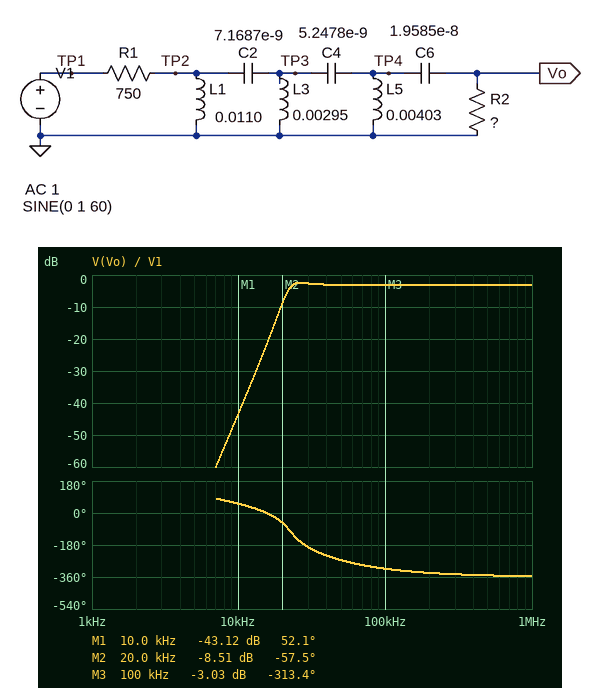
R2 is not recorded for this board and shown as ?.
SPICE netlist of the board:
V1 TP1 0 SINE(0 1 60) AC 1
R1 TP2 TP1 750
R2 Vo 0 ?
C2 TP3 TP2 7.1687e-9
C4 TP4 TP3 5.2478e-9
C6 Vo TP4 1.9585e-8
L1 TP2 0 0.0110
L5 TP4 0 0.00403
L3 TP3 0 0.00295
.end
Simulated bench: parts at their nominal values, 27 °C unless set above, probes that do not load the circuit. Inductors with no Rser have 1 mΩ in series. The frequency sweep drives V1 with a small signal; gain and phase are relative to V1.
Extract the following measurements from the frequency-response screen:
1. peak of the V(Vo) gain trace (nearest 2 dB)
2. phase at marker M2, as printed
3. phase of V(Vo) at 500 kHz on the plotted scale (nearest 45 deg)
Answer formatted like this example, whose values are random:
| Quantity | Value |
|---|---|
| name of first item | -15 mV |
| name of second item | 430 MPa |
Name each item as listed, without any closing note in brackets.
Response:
| Quantity | Value |
|---|---|
| peak of the V(Vo) gain trace | -2 dB |
| phase at marker M2, as printed | -57.5 deg |
| phase of V(Vo) at 500 kHz on the plotted scale | -360 deg |
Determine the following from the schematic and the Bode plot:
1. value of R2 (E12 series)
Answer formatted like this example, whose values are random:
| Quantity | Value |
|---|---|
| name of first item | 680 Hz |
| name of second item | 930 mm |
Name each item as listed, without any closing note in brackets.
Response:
| Quantity | Value |
|---|---|
| value of R2 | 1.8 kΩ |
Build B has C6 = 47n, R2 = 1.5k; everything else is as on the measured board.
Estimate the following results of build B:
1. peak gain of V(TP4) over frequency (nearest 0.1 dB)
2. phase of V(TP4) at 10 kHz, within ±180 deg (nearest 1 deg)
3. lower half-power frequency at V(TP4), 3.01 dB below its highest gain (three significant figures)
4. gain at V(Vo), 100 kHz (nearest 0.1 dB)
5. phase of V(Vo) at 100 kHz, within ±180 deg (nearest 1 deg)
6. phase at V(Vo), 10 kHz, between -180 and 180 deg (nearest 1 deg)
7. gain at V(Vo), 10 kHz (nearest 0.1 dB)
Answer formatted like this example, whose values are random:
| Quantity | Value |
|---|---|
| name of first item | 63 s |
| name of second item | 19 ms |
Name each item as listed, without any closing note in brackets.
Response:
| Quantity | Value |
|---|---|
| peak gain of V(TP4) over frequency | -3.1 dB |
| phase of V(TP4) at 10 kHz, within ±180 deg | 25 deg |
| lower half-power frequency at V(TP4), 3.01 dB below its highest gain | 21.5 kHz |
| gain at V(Vo), 100 kHz | -3.5 dB |
| phase of V(Vo) at 100 kHz, within ±180 deg | 45 deg |
| phase at V(Vo), 10 kHz, between -180 and 180 deg | 38 deg |
| gain at V(Vo), 10 kHz | -42.8 dB |
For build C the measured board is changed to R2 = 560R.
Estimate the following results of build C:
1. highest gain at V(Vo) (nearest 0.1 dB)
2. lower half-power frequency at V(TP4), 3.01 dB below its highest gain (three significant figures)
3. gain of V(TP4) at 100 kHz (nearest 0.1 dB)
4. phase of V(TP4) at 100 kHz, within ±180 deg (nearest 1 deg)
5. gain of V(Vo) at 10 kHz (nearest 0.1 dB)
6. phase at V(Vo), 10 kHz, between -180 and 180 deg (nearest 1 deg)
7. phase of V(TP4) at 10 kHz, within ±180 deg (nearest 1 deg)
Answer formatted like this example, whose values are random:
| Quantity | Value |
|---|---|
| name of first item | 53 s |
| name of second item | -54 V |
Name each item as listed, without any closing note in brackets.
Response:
| Quantity | Value |
|---|---|
| highest gain at V(Vo) | -7.4 dB |
| lower half-power frequency at V(TP4), 3.01 dB below its highest gain | 20.0 kHz |
| gain of V(TP4) at 100 kHz | -7.3 dB |
| phase of V(TP4) at 100 kHz, within ±180 deg | 38 deg |
| gain of V(Vo) at 10 kHz | -45.6 dB |
| phase at V(Vo), 10 kHz, between -180 and 180 deg | 79 deg |
| phase of V(TP4) at 10 kHz, within ±180 deg | 24 deg |
